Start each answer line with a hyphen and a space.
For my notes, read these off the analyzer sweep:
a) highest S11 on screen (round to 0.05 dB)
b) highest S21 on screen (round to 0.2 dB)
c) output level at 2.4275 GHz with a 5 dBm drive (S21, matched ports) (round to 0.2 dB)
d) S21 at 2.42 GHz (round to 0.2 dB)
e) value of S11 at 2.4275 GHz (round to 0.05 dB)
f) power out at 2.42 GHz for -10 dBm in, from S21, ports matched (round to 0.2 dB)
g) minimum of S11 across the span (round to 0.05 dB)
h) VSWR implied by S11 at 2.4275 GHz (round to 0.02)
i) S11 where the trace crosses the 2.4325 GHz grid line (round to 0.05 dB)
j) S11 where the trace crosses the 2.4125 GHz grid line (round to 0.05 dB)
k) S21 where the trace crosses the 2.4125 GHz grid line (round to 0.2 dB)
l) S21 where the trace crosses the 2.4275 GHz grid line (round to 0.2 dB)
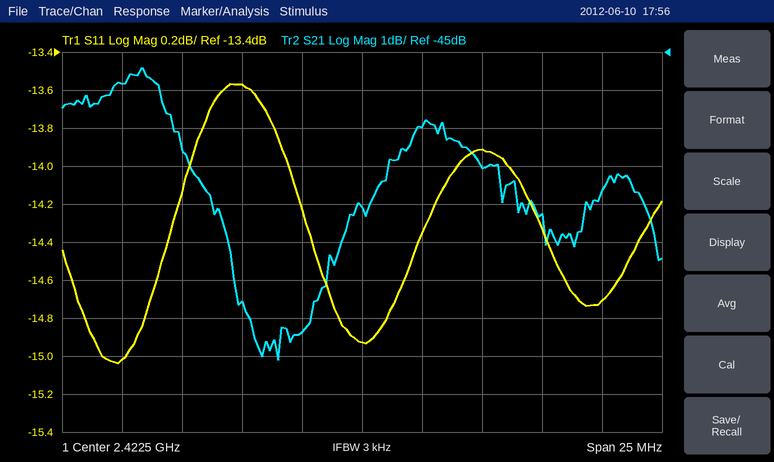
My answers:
- -13.55 dB
- -45.4 dB
- -43.0 dBm
- -52.4 dB
- -13.90 dB
- -62.4 dBm
- -15.05 dB
- 1.50
- -14.70 dB
- -15.00 dB
- -45.8 dB
- -48.0 dB
